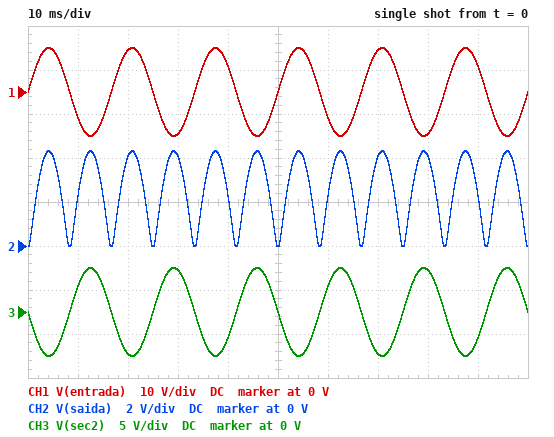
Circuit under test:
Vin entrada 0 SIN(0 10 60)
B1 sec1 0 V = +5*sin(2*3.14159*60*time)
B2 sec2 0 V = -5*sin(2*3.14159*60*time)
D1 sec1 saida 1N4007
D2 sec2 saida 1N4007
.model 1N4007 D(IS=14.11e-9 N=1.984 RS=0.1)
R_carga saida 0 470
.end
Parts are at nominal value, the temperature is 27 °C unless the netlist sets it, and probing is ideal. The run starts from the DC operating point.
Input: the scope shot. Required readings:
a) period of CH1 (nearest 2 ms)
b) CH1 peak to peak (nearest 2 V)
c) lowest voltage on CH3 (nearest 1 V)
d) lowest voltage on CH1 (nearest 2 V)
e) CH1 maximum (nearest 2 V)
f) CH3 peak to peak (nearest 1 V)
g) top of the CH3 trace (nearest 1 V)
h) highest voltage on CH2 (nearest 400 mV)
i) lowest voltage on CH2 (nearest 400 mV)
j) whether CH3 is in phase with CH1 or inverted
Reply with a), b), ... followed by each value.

a) 16 ms
b) 20 V
c) -5 V
d) -10 V
e) 10 V
f) 10 V
g) 5 V
h) 4.4 V
i) 0 V
j) inverted
